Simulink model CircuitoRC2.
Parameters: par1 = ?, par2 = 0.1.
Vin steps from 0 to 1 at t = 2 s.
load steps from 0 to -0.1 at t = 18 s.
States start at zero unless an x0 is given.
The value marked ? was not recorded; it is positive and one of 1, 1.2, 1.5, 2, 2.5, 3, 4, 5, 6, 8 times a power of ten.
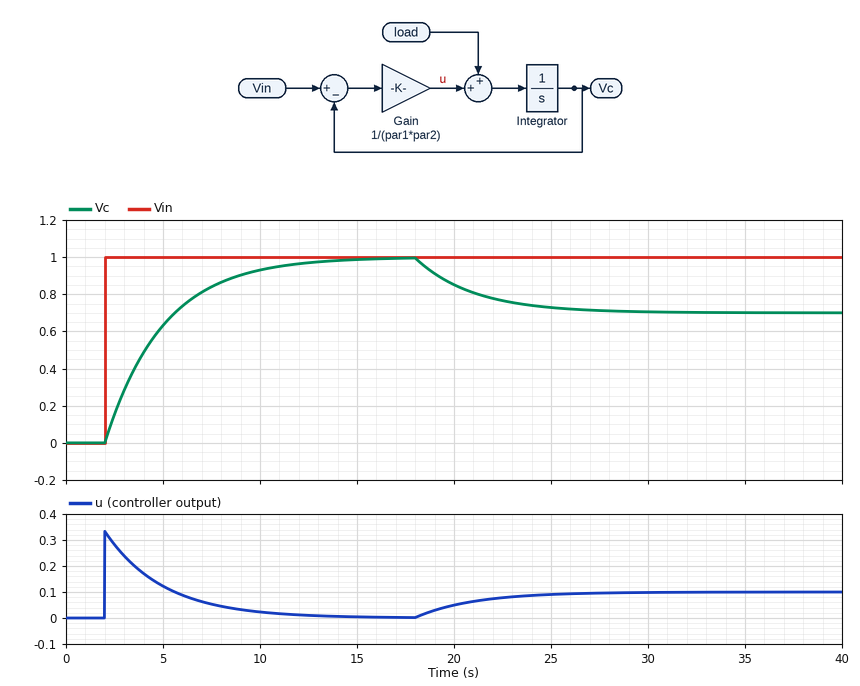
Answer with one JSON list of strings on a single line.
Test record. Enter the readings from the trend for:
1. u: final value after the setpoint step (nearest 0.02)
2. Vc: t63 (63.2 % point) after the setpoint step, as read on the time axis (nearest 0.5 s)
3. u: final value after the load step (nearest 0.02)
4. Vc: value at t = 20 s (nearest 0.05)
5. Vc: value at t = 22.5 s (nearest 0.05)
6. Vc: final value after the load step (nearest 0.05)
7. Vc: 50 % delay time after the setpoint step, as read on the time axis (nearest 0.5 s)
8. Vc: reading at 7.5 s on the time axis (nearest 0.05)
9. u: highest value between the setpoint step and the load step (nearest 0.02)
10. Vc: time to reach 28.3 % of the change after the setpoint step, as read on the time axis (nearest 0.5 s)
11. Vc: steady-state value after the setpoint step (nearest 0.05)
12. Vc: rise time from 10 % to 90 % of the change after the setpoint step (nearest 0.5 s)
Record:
["0.00", "5.0 s", "0.10", "0.85", "0.75", "0.70", "4.0 s", "0.85", "0.34", "3.0 s", "1.00", "6.5 s"]
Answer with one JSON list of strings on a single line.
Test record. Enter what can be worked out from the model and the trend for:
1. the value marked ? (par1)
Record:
["30"]
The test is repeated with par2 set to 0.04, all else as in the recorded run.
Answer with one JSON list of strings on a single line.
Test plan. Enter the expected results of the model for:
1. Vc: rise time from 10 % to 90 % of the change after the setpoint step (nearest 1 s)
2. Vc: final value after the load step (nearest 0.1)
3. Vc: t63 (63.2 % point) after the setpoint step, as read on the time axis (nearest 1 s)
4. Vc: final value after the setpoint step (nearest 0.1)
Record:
["3 s", "0.9", "3 s", "1.0"]
